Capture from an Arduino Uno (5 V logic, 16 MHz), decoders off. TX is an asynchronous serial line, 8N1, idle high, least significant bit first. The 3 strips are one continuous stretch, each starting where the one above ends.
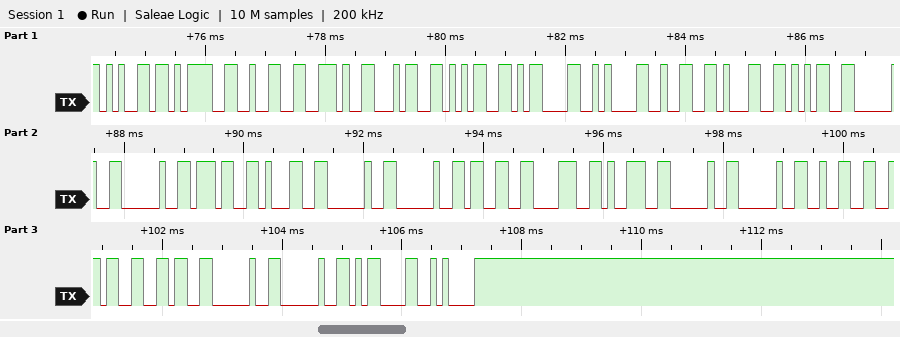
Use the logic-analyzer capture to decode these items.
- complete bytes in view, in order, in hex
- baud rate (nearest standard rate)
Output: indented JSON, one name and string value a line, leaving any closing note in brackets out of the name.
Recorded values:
{
  "complete bytes in view, in order, in hex": "65 3D 32 2E 34 35 0D 0A 32 31 35 20 20 37 31 20 20 33 38 39 20 20 32 36 36 20 20 0D 0A",
  "baud rate": "9600 baud"
}
